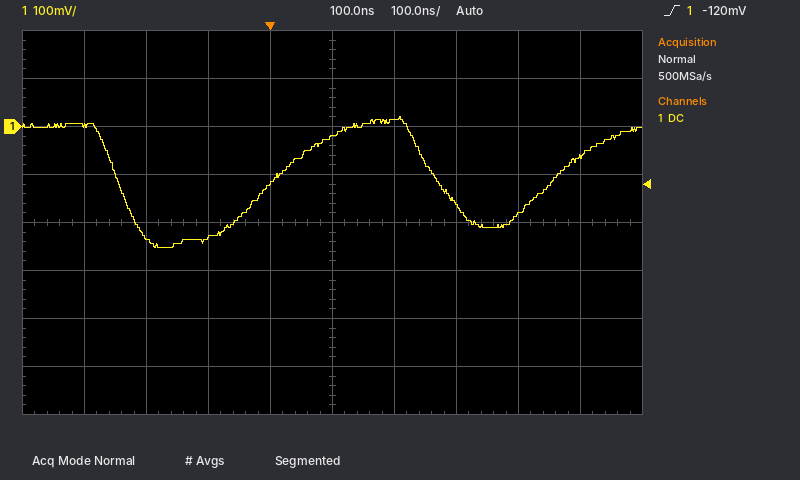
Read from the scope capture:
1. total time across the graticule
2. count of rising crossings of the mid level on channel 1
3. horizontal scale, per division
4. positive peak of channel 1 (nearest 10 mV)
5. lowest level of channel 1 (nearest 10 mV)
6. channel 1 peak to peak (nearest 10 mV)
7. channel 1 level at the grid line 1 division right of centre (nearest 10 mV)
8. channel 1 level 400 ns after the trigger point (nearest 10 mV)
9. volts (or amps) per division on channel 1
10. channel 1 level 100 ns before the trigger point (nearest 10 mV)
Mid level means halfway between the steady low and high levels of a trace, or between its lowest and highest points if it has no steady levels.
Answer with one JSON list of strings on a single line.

["1 µs", "2", "100 ns", "20 mV", "-250 mV", "270 mV", "10 mV", "-180 mV", "100 mV", "-230 mV"]
